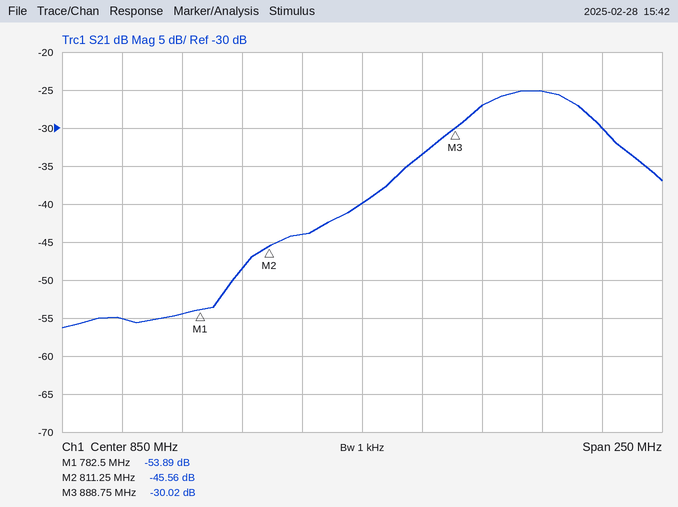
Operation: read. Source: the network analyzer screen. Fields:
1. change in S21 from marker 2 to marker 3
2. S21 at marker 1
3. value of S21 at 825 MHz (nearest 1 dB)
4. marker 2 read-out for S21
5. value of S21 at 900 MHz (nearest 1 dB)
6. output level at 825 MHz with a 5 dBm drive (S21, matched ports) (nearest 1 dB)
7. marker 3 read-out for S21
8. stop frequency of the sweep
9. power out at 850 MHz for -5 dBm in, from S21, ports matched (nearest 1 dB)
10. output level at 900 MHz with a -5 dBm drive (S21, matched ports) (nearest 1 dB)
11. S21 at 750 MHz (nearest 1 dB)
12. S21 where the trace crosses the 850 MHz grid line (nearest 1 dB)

15.54 dB
-53.89 dB
-44 dB
-45.56 dB
-27 dB
-39 dBm
-30.02 dB
975 MHz
-45 dBm
-32 dBm
-55 dB
-40 dB
